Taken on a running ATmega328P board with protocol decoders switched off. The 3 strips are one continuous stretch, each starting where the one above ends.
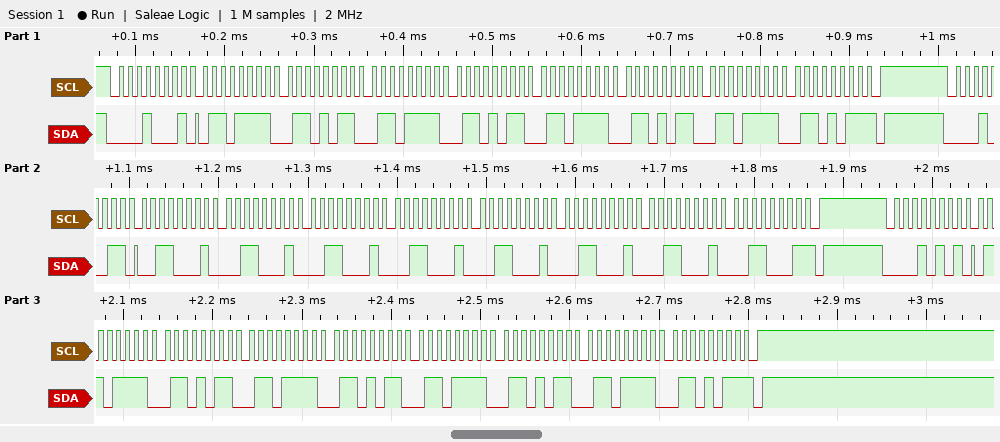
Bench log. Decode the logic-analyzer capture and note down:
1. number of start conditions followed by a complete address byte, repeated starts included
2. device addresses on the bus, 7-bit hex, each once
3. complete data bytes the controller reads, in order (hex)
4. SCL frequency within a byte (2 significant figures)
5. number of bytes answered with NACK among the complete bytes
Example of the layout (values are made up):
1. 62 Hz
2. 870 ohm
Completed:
1. 3
2. 0x08 0x09 0x0A
3. 6F 6B 6F 6B 6F 6B 6F 6B 31 31 31 31 31 31 31 31 6F 6B 6F 6B 6F 6B 6F 6B
4. 100 kHz
5. 3
